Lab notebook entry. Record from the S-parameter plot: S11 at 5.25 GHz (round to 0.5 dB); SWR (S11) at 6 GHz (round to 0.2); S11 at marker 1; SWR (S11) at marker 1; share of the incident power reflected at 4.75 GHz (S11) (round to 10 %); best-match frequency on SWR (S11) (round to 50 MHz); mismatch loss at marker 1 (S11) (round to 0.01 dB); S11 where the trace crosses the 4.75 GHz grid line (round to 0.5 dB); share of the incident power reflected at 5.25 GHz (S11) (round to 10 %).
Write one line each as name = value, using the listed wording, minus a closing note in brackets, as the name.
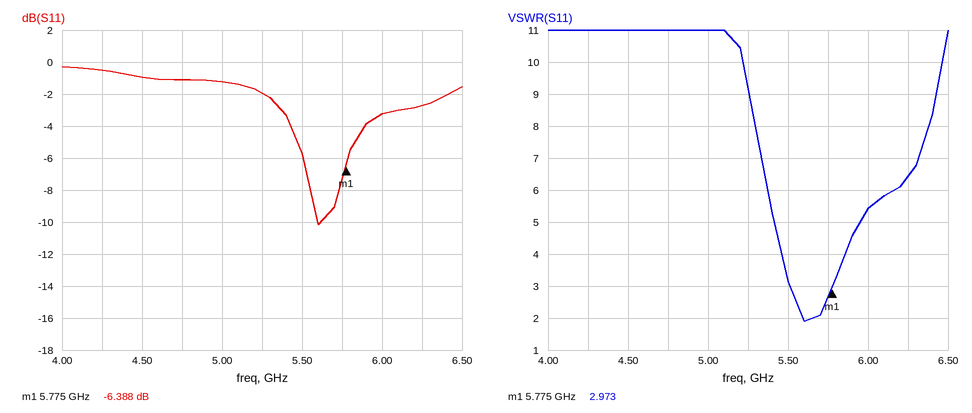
S11 at 5.25 GHz = -2.0 dB
SWR (S11) at 6 GHz = 5.4
S11 at marker 1 = -6.388 dB
SWR (S11) at marker 1 = 2.973
share of the incident power reflected at 4.75 GHz (S11) = 80 %
best-match frequency on SWR (S11) = 5.60 GHz
mismatch loss at marker 1 (S11) = 1.13 dB
S11 where the trace crosses the 4.75 GHz grid line = -1.0 dB
share of the incident power reflected at 5.25 GHz (S11) = 60 %
